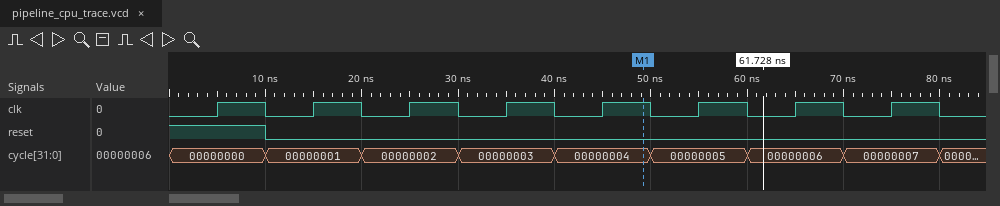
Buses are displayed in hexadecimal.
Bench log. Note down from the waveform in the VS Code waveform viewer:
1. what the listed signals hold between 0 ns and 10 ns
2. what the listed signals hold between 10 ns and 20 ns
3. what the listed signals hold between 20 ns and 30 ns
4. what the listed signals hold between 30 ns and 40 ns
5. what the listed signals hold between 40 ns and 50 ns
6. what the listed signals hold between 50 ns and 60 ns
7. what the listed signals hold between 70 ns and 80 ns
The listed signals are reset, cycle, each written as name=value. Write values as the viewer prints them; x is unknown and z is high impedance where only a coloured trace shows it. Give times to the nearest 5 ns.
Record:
reset=1, cycle=00000000
reset=0, cycle=00000001
reset=0, cycle=00000002
reset=0, cycle=00000003
reset=0, cycle=00000004
reset=0, cycle=00000005
reset=0, cycle=00000007
